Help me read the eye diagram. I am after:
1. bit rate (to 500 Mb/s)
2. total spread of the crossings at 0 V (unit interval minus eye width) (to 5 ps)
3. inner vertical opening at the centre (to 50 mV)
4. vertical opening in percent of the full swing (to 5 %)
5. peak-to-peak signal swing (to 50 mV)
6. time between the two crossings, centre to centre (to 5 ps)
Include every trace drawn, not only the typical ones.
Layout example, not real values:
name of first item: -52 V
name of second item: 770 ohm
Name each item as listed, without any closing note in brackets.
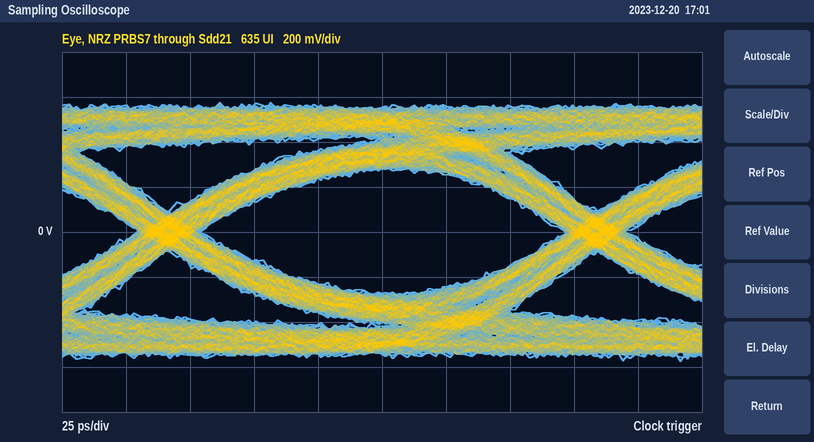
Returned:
bit rate: 6.0 Gb/s
total spread of the crossings at 0 V (unit interval minus eye width): 25 ps
inner vertical opening at the centre: 550 mV
vertical opening in percent of the full swing: 50 %
peak-to-peak signal swing: 1.15 V
time between the two crossings, centre to centre: 165 ps
